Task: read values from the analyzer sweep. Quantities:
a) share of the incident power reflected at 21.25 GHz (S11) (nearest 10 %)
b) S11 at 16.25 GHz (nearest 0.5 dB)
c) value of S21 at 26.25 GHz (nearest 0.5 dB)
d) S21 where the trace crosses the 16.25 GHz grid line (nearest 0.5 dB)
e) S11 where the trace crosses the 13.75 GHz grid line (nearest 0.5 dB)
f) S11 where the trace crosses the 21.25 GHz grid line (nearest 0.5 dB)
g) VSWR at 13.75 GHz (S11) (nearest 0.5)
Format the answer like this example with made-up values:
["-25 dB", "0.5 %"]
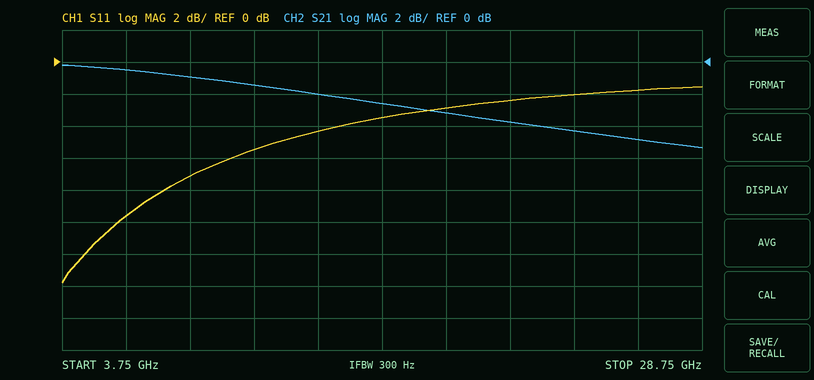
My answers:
["60 %", "-3.5 dB", "-5.0 dB", "-2.5 dB", "-4.5 dB", "-2.5 dB", "4.0"]
